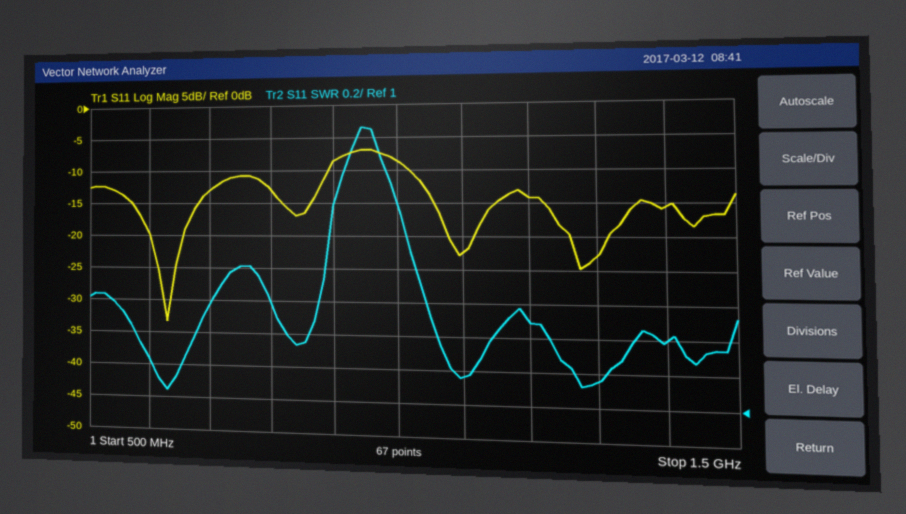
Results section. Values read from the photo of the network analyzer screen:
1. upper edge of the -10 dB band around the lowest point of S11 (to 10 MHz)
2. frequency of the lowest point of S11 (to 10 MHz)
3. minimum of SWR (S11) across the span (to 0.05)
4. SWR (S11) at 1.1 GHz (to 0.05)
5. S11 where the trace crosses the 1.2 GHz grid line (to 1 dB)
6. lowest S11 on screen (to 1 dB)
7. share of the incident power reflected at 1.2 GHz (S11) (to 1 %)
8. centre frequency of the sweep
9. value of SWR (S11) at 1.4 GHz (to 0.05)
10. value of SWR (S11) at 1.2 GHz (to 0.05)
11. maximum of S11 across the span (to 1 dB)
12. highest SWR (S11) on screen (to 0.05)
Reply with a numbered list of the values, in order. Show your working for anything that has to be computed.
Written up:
1. 890 MHz
2. 630 MHz
3. 1.05
4. 1.15
5. -14 dB
6. -33 dB
7. 10^(-14/10) ≈ 4 %
8. 1 GHz
9. 1.40
10. 1.50
11. -7 dB
12. 2.65
